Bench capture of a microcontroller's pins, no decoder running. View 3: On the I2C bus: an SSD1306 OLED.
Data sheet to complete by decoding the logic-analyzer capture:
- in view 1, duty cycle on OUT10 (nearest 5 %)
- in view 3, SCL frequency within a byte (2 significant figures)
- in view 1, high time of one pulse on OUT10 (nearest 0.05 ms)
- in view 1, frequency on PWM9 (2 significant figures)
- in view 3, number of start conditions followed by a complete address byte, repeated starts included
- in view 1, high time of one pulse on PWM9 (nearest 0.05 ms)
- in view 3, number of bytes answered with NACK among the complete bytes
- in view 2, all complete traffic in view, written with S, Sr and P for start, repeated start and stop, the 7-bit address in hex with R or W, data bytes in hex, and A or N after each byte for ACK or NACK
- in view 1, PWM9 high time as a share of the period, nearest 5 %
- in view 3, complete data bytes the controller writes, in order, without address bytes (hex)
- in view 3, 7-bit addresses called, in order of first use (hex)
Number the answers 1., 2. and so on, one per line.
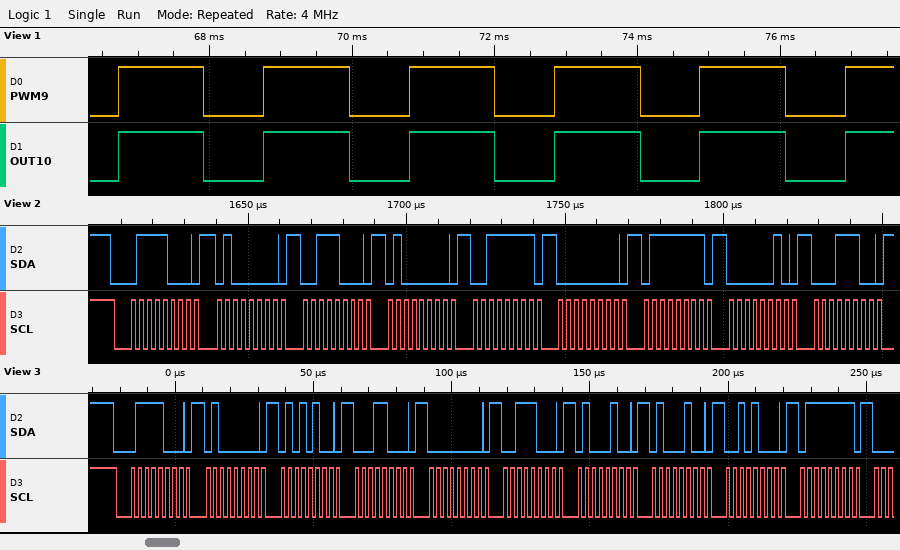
1. 60 %
2. 400 kHz
3. 1.20 ms
4. 490 Hz
5. 1
6. 1.20 ms
7. 0
8. S 3CW A 40 A 38 A 40 A 3F A 00 A 7F A 02 A 1C A
9. 60 %
10. 40 54 18 00 38 44 44 28 7F
11. 0x3C
